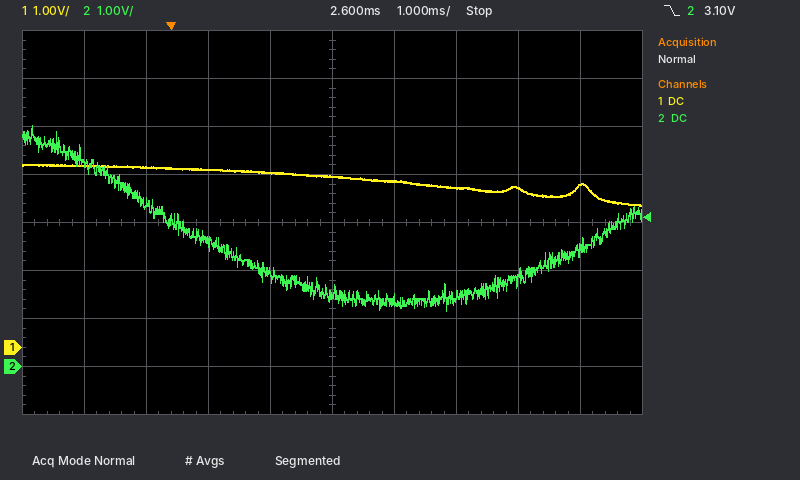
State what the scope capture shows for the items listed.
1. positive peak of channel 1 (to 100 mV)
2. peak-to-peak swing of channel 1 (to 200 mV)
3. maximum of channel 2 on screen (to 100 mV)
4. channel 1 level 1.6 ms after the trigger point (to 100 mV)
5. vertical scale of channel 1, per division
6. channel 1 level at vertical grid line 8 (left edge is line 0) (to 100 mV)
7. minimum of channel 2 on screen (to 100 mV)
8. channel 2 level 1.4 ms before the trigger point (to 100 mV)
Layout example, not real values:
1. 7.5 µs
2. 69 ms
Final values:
1. 3.8 V
2. 800 mV
3. 5.0 V
4. 3.6 V
5. 1 V
6. 3.3 V
7. 1.2 V
8. 4.2 V
